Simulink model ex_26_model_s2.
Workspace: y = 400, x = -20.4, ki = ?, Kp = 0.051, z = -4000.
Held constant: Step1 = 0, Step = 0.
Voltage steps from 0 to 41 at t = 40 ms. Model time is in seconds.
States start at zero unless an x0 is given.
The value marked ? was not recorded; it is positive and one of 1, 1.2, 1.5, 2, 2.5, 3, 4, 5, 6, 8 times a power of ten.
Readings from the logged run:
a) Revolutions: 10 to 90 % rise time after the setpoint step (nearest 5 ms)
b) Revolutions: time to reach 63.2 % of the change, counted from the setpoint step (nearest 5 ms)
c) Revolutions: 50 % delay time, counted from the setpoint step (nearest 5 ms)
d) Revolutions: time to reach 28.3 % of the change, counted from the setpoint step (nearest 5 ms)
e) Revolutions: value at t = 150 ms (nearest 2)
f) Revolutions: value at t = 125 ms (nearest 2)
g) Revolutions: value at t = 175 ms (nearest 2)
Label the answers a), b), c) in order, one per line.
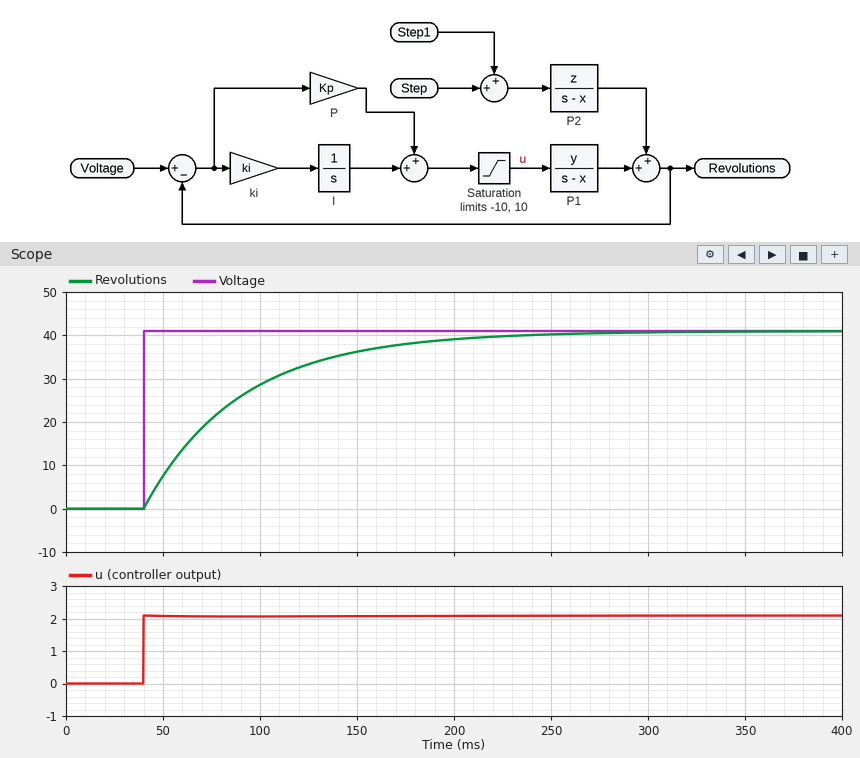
a) 115 ms
b) 50 ms
c) 35 ms
d) 15 ms
e) 36
f) 34
g) 38
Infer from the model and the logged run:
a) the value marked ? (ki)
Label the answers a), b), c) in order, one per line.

a) 1
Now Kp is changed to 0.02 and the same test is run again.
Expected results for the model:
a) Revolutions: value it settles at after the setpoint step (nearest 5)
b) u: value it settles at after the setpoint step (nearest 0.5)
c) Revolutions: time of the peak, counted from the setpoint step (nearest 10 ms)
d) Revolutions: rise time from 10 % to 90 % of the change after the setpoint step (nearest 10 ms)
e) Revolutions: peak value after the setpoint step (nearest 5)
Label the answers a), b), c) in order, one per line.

a) 40
b) 2.0
c) 200 ms
d) 100 ms
e) 45
